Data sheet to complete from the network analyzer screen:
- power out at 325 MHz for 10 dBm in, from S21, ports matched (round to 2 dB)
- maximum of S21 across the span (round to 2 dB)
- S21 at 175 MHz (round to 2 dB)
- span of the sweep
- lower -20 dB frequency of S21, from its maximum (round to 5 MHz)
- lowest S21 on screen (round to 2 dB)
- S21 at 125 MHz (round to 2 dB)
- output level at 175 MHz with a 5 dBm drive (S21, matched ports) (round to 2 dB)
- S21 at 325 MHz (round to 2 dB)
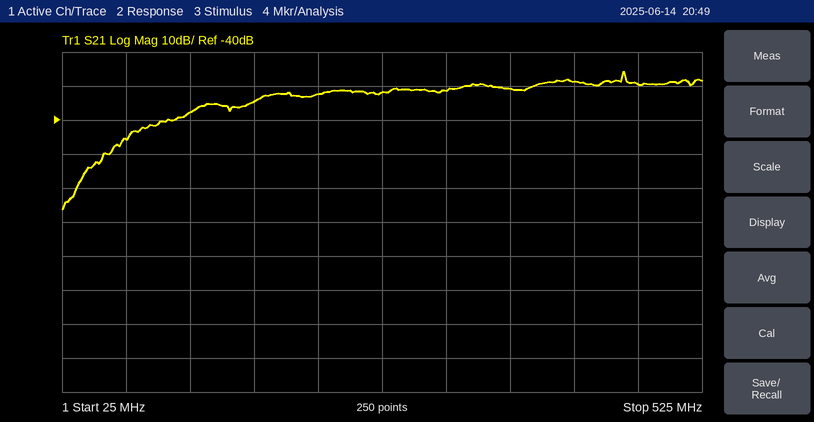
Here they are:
-22 dBm
-26 dB
-34 dB
500 MHz
75 MHz
-66 dB
-38 dB
-30 dBm
-32 dB
